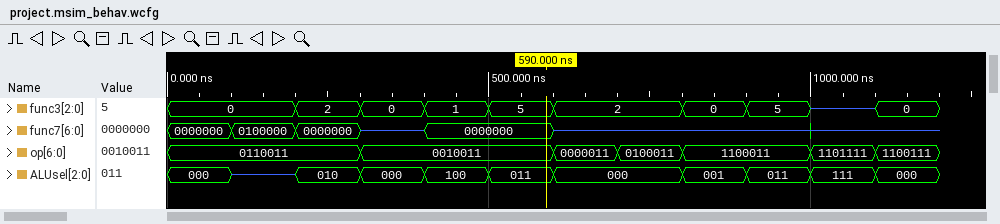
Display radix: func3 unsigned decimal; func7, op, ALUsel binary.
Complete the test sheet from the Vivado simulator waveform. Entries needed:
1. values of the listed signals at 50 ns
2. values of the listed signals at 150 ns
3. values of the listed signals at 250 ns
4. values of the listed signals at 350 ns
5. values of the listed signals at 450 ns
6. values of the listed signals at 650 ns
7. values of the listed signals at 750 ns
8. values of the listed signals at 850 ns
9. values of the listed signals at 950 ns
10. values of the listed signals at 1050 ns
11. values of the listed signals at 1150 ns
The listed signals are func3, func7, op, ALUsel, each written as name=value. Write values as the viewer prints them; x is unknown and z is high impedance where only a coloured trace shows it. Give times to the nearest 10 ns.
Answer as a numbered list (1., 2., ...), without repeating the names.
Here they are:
1. func3=0, func7=0000000, op=0110011, ALUsel=000
2. func3=0, func7=0100000, op=0110011, ALUsel=z
3. func3=2, func7=0000000, op=0110011, ALUsel=010
4. func3=0, func7=z, op=0010011, ALUsel=000
5. func3=1, func7=0000000, op=0010011, ALUsel=100
6. func3=2, func7=z, op=0000011, ALUsel=000
7. func3=2, func7=z, op=0100011, ALUsel=000
8. func3=0, func7=z, op=1100011, ALUsel=001
9. func3=5, func7=z, op=1100011, ALUsel=011
10. func3=z, func7=z, op=1101111, ALUsel=111
11. func3=0, func7=z, op=1100111, ALUsel=000
